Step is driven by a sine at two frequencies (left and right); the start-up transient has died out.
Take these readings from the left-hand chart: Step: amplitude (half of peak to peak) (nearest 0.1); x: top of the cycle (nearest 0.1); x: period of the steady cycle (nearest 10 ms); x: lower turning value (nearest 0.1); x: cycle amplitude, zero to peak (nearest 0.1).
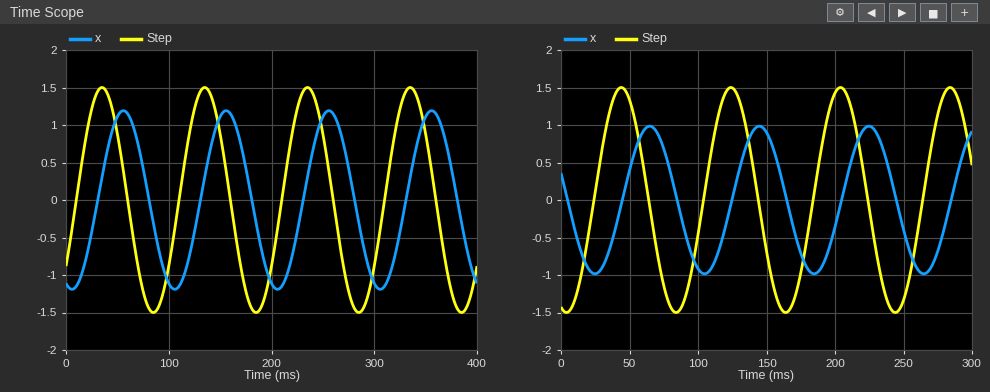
1.5
1.2
100 ms
-1.2
1.2
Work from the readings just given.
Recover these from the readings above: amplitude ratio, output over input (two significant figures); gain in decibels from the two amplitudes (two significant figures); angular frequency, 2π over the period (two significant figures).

0.80
-1.9 dB
0.063 rad/ms
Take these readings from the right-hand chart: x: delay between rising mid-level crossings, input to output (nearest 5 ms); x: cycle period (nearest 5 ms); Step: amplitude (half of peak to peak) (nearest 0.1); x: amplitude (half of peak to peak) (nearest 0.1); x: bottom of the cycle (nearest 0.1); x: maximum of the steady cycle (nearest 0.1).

20 ms
80 ms
1.5
1.0
-1.0
1.0
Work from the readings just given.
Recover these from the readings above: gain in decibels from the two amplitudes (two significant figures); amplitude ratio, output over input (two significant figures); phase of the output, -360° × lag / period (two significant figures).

-3.5 dB
0.67
-90°
